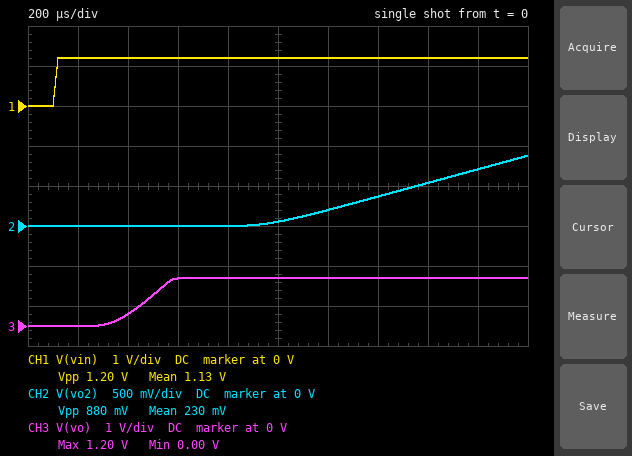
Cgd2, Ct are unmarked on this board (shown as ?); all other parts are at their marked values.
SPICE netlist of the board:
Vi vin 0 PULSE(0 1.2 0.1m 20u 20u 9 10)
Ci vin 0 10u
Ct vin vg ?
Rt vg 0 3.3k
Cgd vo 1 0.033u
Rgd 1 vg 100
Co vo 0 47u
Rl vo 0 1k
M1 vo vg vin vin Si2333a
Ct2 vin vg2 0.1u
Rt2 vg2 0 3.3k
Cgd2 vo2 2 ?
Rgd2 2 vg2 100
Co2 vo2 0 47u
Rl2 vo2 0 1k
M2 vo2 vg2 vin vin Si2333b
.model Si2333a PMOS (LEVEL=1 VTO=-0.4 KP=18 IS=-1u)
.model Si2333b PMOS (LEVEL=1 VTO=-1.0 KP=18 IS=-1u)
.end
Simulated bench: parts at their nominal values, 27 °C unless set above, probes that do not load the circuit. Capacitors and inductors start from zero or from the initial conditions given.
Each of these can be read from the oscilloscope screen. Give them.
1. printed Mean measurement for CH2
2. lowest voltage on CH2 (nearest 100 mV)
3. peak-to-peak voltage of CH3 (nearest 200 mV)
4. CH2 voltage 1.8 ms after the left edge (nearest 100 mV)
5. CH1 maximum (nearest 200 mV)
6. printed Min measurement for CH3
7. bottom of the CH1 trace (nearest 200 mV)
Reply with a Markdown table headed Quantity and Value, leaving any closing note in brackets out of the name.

| Quantity | Value |
|---|---|
| printed Mean measurement for CH2 | 230 mV |
| lowest voltage on CH2 | 0 V |
| peak-to-peak voltage of CH3 | 1.2 V |
| CH2 voltage 1.8 ms after the left edge | 700 mV |
| CH1 maximum | 1.2 V |
| printed Min measurement for CH3 | 0.00 V |
| bottom of the CH1 trace | 0 V |
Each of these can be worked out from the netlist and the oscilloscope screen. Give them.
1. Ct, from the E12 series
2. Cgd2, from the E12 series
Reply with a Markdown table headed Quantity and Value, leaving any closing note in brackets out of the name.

| Quantity | Value |
|---|---|
| Ct, from the E12 series | 150 nF |
| Cgd2, from the E12 series | 47 nF |
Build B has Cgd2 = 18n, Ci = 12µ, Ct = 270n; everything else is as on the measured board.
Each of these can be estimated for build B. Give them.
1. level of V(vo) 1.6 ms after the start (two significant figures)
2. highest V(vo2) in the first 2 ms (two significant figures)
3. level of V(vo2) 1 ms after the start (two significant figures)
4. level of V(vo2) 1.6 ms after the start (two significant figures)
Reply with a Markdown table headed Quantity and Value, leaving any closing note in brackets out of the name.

| Quantity | Value |
|---|---|
| level of V(vo) 1.6 ms after the start | 1.2 V |
| highest V(vo2) in the first 2 ms | 1.2 V |
| level of V(vo2) 1 ms after the start | 140 mV |
| level of V(vo2) 1.6 ms after the start | 1.1 V |
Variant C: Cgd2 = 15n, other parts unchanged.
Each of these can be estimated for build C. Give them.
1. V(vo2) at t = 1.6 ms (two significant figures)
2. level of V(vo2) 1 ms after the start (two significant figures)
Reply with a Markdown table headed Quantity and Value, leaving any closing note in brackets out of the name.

| Quantity | Value |
|---|---|
| V(vo2) at t = 1.6 ms | 1.2 V |
| level of V(vo2) 1 ms after the start | 160 mV |
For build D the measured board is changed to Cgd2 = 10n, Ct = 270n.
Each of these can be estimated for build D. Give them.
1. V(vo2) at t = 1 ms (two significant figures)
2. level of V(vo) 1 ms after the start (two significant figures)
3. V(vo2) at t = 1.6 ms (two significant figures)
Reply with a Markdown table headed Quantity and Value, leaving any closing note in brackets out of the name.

| Quantity | Value |
|---|---|
| V(vo2) at t = 1 ms | 200 mV |
| level of V(vo) 1 ms after the start | 1.2 V |
| V(vo2) at t = 1.6 ms | 1.2 V |
